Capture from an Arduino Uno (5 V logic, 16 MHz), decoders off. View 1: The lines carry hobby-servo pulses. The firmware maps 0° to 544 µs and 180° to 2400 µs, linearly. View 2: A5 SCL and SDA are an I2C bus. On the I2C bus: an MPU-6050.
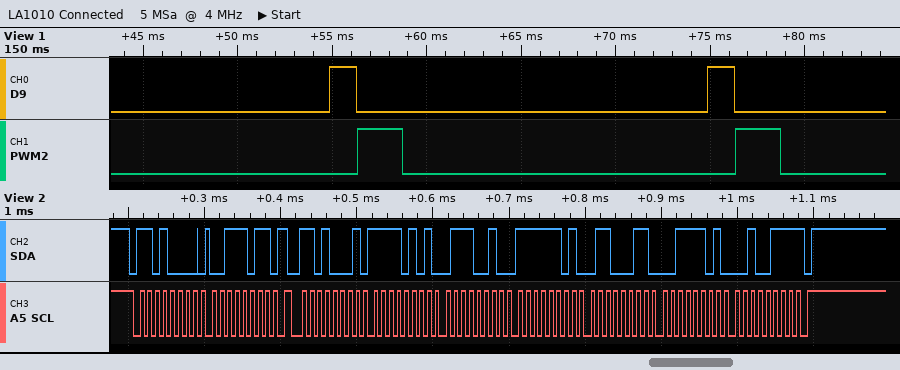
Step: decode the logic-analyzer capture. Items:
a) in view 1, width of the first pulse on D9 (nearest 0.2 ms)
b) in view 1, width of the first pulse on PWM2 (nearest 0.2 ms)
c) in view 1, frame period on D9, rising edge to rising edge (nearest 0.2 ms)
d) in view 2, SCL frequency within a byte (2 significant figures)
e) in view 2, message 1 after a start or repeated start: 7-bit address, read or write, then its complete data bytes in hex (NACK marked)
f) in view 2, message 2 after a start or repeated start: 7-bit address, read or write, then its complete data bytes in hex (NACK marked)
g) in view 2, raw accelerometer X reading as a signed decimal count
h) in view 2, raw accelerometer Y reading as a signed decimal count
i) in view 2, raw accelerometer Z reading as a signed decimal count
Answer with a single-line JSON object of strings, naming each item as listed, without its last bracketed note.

{"in view 1, width of the first pulse on D9": "1.4 ms", "in view 1, width of the first pulse on PWM2": "2.4 ms", "in view 1, frame period on D9, rising edge to rising edge": "20.0 ms", "in view 2, SCL frequency within a byte": "100 kHz", "in view 2, message 1 after a start or repeated start: 7-bit address, read or write, then its complete data bytes in hex": "0x68 write: 3B", "in view 2, message 2 after a start or repeated start: 7-bit address, read or write, then its complete data bytes in hex": "0x68 read: F5 72 FD 63 3D 27 NACK", "in view 2, raw accelerometer X reading as a signed decimal count": "-2702", "in view 2, raw accelerometer Y reading as a signed decimal count": "-669", "in view 2, raw accelerometer Z reading as a signed decimal count": "15655"}
